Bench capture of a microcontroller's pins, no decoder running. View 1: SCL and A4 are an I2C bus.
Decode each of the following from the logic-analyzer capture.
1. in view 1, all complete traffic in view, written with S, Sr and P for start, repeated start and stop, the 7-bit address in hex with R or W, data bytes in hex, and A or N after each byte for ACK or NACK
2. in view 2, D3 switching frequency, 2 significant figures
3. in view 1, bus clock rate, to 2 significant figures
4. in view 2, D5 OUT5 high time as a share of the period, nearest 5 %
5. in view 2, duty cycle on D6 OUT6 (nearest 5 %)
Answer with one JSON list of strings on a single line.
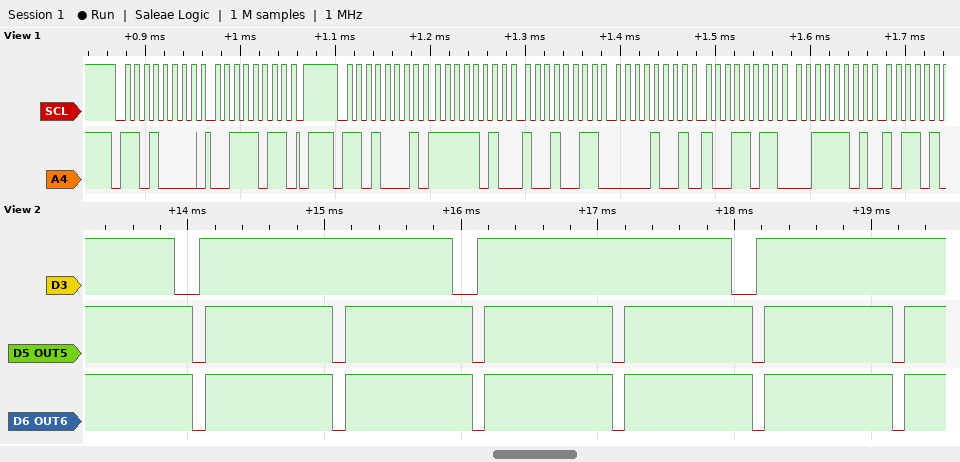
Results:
["S 68W A 3B A P S 68R A FA A 93 A 09 A 9B A 3D A", "490 Hz", "100 kHz", "90 %", "90 %"]
